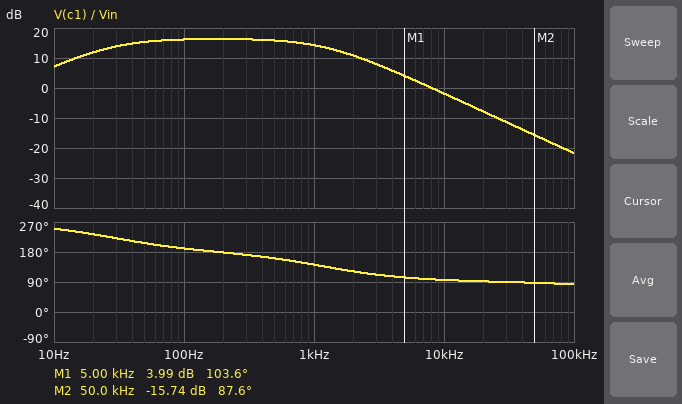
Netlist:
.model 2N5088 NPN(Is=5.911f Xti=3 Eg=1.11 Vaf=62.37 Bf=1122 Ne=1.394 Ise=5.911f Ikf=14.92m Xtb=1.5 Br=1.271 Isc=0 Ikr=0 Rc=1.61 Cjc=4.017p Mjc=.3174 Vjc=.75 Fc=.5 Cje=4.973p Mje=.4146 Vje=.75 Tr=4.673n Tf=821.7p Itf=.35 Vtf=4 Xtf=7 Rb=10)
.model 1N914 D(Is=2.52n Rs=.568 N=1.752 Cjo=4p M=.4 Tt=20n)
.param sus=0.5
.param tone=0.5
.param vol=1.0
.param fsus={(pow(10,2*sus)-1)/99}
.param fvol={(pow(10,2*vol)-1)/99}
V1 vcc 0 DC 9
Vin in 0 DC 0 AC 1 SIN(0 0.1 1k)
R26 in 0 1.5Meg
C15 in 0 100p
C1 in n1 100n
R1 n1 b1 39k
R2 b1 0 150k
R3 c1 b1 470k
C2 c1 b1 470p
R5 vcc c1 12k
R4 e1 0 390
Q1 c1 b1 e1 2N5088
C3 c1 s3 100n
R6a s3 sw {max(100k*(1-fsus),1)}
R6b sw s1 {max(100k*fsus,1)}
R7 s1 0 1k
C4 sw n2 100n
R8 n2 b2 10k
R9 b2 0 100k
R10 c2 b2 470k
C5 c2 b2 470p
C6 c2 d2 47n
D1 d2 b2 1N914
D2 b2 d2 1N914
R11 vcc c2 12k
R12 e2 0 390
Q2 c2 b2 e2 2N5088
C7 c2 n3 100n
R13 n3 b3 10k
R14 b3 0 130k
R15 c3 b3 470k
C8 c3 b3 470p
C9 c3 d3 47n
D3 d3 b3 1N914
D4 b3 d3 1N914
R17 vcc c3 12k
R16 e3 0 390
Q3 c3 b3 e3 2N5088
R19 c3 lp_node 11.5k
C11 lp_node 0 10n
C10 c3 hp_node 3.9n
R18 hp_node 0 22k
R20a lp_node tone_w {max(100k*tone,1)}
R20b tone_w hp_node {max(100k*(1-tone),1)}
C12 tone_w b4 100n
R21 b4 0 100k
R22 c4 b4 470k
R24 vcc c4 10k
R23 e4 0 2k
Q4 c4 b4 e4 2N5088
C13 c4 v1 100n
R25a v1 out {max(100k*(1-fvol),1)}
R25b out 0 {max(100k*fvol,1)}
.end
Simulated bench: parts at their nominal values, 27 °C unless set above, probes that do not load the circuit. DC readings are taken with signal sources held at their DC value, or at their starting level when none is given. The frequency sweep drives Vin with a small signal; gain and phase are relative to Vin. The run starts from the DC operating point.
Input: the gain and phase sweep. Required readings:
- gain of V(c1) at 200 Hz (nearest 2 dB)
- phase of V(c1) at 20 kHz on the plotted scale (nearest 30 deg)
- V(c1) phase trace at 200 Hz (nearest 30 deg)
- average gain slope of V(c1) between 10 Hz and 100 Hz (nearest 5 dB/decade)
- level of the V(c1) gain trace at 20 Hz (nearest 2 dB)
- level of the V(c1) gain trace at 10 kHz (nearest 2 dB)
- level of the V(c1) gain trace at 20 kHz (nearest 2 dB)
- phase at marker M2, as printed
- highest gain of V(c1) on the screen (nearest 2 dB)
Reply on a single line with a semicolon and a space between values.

16 dB; 90 deg; 180 deg; 10 dB/decade; 12 dB; -2 dB; -8 dB; 87.6 deg; 16 dB
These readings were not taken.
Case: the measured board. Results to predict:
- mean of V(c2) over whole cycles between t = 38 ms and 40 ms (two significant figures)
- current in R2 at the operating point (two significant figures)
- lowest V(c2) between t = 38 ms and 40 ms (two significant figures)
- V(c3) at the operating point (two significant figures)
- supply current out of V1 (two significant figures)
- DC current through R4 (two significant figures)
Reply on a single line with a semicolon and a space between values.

4.7 V; 5.4 µA; 4.5 V; 4.0 V; 1.5 mA; 430 µA
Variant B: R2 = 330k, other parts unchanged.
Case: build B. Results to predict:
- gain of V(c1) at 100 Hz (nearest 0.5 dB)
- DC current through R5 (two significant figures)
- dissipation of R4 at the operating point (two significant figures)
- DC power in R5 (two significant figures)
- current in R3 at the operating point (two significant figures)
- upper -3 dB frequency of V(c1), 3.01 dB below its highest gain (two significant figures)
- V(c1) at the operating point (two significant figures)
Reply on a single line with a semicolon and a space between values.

16.5 dB; 540 µA; 110 µW; 3.5 mW; 3.5 µA; 1.2 kHz; 2.5 V
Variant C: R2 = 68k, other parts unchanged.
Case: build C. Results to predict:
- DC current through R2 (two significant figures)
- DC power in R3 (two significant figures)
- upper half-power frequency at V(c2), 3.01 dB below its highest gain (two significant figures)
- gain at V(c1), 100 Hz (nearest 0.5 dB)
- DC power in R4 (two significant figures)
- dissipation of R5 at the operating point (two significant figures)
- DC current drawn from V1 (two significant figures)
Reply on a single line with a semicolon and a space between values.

11 µA; 58 µW; 1.0 kHz; 15.0 dB; 23 µW; 780 µW; 1.3 mA
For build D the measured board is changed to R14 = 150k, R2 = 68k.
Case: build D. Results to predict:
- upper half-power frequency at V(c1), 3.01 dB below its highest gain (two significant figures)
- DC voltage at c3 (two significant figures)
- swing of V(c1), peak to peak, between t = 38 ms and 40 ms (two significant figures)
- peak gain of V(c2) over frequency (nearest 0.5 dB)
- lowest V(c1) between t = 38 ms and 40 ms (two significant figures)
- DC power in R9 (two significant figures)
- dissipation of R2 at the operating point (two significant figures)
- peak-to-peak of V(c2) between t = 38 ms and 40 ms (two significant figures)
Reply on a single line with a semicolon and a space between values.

1.4 kHz; 3.7 V; 950 mV; 13.5 dB; 5.5 V; 6.0 µW; 7.7 µW; 460 mV
